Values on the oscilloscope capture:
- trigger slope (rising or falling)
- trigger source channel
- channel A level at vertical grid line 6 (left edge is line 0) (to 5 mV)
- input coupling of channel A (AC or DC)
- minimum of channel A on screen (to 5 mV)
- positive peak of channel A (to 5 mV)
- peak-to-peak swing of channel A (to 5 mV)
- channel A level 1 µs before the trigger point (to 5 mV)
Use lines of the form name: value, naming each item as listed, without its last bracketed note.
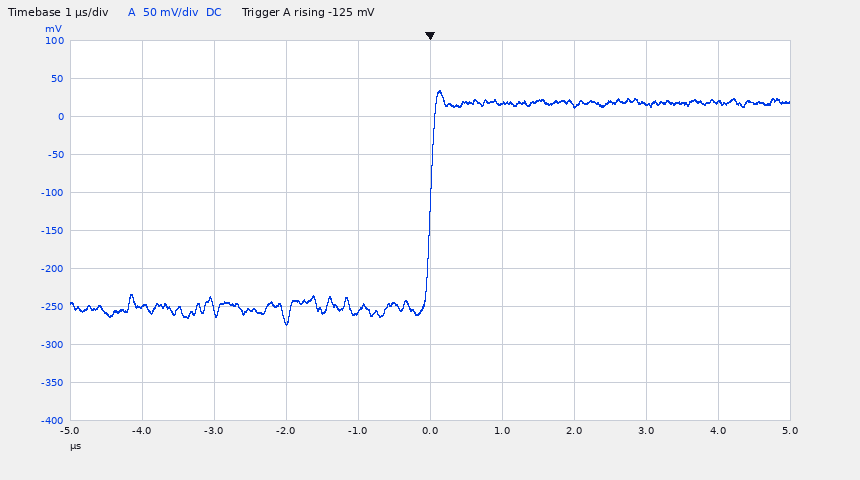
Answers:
trigger slope: rising
trigger source channel: channel A
channel A level at vertical grid line 6 (left edge is line 0): 15 mV
input coupling of channel A: DC
minimum of channel A on screen: -275 mV
positive peak of channel A: 35 mV
peak-to-peak swing of channel A: 310 mV
channel A level 1 µs before the trigger point: -255 mV
